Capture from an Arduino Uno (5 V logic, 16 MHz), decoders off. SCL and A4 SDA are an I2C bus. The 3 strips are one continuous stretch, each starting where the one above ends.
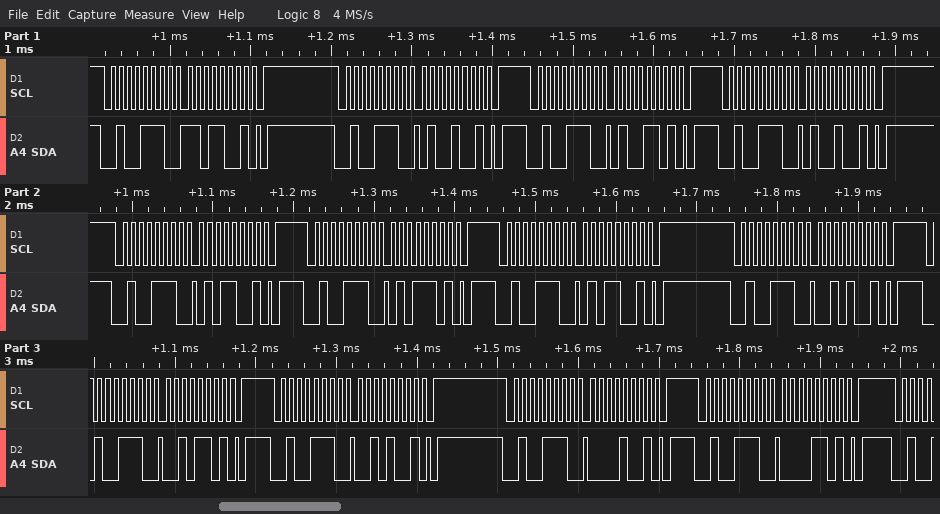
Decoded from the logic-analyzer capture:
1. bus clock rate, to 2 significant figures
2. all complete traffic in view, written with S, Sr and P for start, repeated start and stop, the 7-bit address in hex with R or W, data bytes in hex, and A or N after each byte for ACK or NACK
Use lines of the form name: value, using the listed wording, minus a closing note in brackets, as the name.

bus clock rate, to 2 significant figures: 100 kHz
all complete traffic in view, written with S, Sr and P for start, repeated start and stop, the 7-bit address in hex with R or W, data bytes in hex, and A or N after each byte for ACK or NACK: S 27W A D9 A P S 27W A 49 A P S 27W A 4D A P S 27W A 49 A P S 27W A 59 A P S 27W A 5D A P S 27W A 59 A P S 27W A 29 A P S 27W A 2D A P S 27W A 29 A P S 27W A 09 A P S 27W A 0D A P
